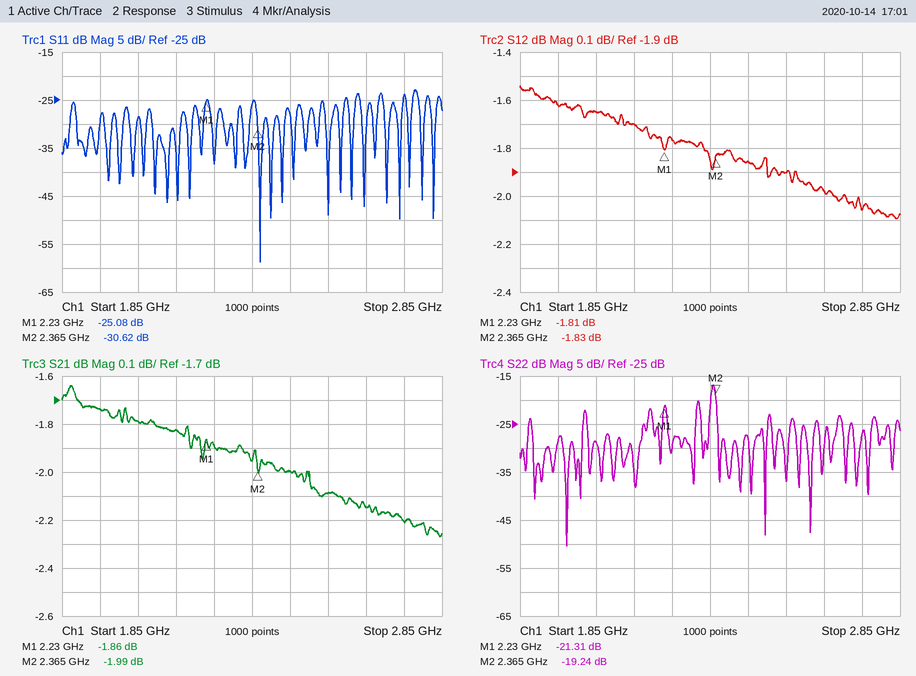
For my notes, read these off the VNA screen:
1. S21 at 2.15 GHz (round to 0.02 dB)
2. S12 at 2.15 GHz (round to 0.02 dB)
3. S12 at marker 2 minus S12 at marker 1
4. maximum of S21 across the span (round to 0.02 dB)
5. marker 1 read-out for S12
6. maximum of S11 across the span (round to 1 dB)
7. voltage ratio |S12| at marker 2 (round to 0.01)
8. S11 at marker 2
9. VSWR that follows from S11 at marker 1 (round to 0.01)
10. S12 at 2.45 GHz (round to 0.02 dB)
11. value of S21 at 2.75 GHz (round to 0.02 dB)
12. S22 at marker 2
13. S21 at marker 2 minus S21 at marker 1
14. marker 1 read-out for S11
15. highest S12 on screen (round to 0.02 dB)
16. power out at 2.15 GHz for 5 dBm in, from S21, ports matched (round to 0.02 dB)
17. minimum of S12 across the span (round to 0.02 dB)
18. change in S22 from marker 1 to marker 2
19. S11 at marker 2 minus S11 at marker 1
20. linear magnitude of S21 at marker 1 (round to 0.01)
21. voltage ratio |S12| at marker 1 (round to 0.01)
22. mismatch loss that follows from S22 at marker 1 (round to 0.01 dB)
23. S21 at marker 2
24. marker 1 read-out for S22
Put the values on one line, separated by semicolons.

-1.82 dB; -1.70 dB; -0.02 dB; -1.64 dB; -1.81 dB; -23 dB; 0.81; -30.62 dB; 1.12; -1.86 dB; -2.20 dB; -19.24 dB; -0.13 dB; -25.08 dB; -1.54 dB; 3.18 dBm; -2.10 dB; 2.07 dB; -5.54 dB; 0.81; 0.81; 0.03 dB; -1.99 dB; -21.31 dB
